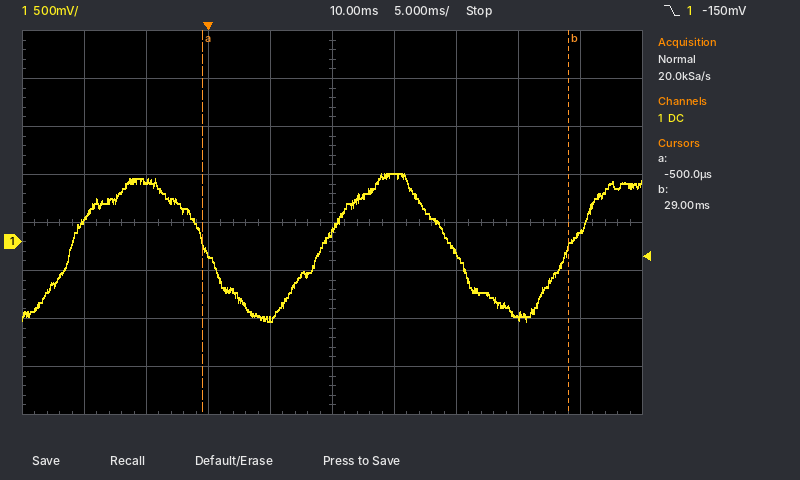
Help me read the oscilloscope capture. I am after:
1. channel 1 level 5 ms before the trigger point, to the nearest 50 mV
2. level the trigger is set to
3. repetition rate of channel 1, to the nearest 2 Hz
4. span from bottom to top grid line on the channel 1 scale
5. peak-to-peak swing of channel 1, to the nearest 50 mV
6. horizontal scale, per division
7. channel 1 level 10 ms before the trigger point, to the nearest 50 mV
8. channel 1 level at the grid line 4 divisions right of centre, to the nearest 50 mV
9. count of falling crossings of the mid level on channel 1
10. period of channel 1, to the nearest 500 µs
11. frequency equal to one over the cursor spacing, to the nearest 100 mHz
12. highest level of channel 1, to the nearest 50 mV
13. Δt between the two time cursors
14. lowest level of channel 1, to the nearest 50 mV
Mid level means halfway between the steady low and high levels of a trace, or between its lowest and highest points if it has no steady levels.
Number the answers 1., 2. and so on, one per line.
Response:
1. 650 mV
2. -150 mV
3. 50 Hz
4. 4 V
5. 1.55 V
6. 5 ms
7. 250 mV
8. 100 mV
9. 2
10. 20.0 ms
11. 33.9 Hz
12. 700 mV
13. 29.5 ms
14. -850 mV
